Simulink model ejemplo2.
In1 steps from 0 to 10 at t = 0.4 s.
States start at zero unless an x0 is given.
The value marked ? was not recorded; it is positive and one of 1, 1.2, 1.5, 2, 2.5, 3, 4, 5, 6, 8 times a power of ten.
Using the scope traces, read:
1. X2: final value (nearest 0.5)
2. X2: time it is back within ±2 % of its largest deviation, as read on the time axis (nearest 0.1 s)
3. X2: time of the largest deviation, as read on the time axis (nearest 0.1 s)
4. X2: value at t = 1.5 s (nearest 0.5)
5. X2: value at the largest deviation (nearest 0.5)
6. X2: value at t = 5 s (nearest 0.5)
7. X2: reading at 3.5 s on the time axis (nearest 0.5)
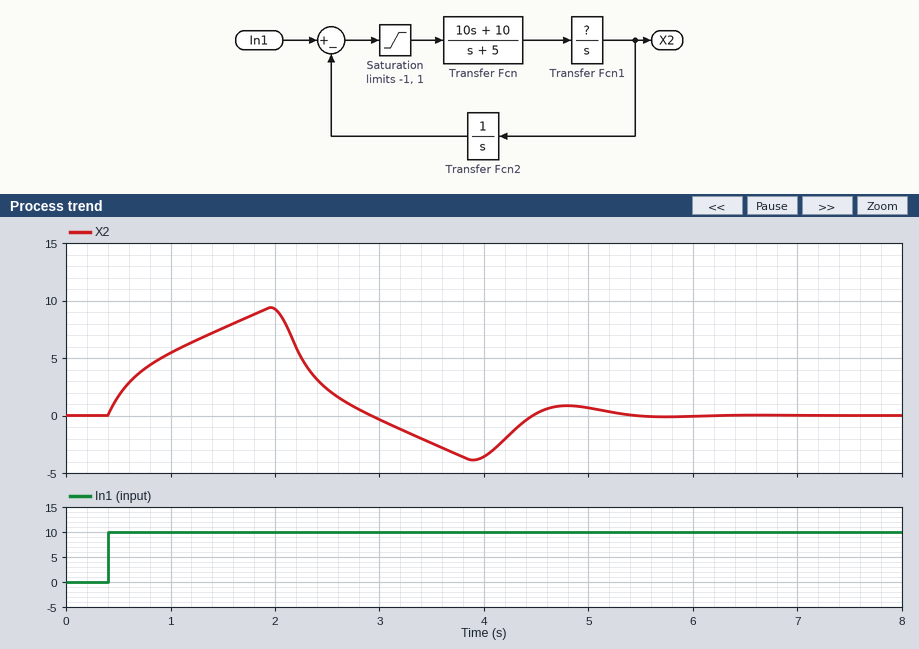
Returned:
0.0
5.3 s
2.0 s
7.5
9.5
0.5
-2.5
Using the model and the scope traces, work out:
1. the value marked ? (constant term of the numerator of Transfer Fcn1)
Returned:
2
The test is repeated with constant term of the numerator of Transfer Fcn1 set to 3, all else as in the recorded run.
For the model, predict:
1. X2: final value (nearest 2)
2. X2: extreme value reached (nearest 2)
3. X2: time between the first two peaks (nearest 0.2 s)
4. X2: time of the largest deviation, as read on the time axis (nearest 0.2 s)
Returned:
0
12
2.0 s
1.6 s
